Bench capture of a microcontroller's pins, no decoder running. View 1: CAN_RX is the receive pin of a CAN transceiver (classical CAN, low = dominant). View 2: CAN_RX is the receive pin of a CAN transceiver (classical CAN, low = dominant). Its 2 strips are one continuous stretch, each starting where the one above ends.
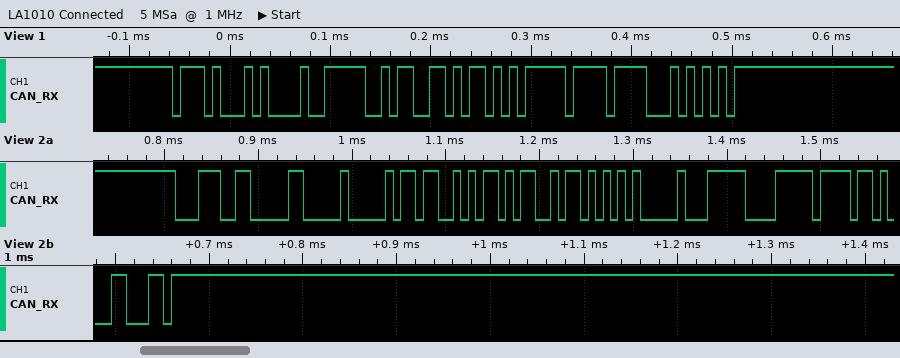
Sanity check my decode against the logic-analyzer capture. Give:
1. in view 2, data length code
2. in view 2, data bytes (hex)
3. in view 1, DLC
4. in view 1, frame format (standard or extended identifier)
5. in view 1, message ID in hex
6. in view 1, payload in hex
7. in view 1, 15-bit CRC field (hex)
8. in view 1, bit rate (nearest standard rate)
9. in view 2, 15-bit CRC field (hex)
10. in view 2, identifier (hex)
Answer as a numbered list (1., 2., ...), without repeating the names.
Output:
1. 8
2. 00 D9 5A CB 55 00 F8 FF
3. 4
4. standard
5. 0x745
6. FA CD 6A FF
7. 0x5E2A
8. 125 kbit/s
9. 0x5A31
10. 0x1CC
